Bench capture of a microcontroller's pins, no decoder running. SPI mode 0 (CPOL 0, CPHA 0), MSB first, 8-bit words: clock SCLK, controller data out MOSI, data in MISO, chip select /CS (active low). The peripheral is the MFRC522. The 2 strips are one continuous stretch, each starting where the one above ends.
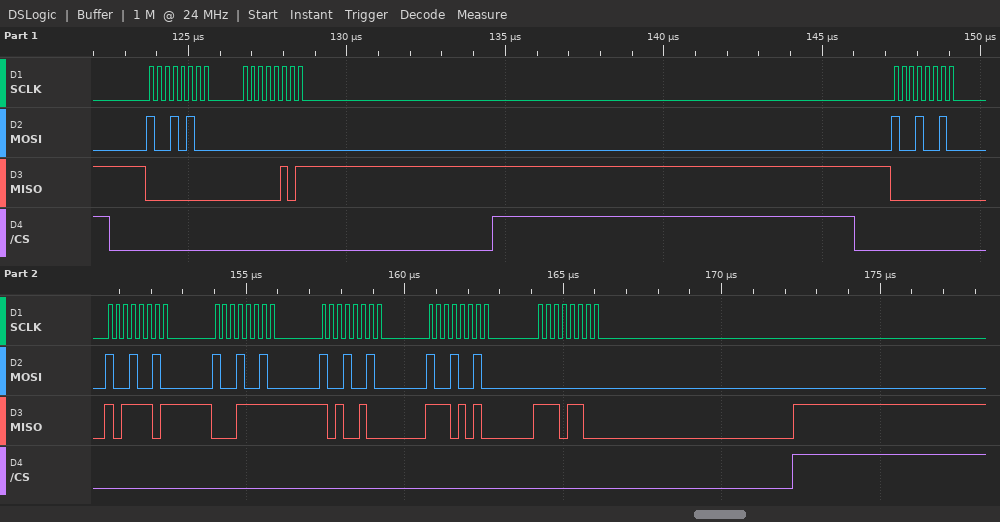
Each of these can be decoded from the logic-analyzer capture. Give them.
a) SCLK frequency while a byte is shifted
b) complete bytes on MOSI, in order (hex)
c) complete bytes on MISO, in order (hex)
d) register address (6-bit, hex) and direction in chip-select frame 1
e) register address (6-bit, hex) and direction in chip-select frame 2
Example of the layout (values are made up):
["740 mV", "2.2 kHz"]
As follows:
["4 MHz", "94 00 92 92 92 92 92 00", "00 05 00 BD 1F A4 EA EC", "0x0A read", "0x09 read"]
